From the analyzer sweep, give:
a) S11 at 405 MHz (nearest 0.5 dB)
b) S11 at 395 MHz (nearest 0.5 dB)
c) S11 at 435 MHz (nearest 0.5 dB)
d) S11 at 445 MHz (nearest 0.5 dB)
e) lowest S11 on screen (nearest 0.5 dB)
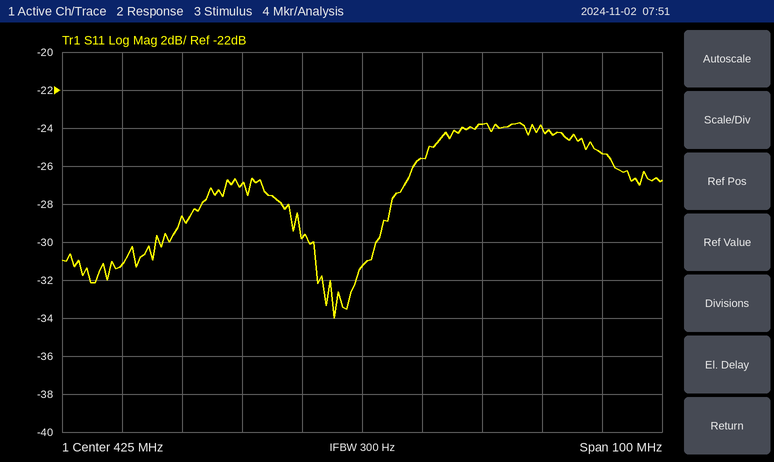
-27.0 dB
-28.5 dB
-25.5 dB
-24.0 dB
-34.0 dB
